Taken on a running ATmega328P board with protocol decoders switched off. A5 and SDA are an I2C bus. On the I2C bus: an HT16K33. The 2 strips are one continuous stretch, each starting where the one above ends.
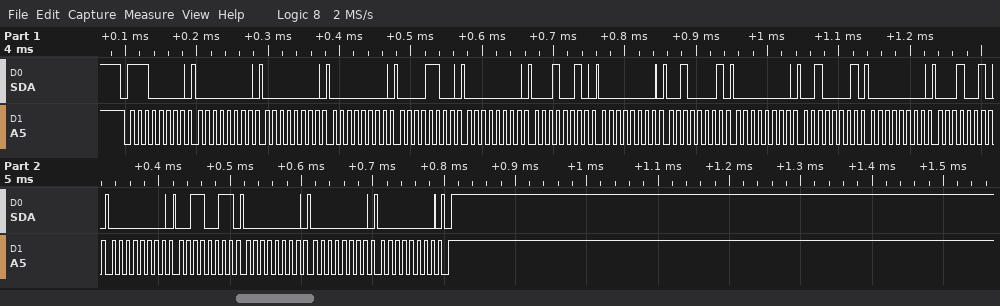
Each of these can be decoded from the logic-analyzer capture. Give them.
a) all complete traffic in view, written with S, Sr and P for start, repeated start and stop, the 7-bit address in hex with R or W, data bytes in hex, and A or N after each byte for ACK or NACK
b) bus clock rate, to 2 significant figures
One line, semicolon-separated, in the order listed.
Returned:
S 70W A 00 A 00 A 00 A 0C A 00 A 12 A 00 A 21 A 00 A 21 A 00 A 12 A 00 A 33 A 00 A 00 A 00 A P; 100 kHz
